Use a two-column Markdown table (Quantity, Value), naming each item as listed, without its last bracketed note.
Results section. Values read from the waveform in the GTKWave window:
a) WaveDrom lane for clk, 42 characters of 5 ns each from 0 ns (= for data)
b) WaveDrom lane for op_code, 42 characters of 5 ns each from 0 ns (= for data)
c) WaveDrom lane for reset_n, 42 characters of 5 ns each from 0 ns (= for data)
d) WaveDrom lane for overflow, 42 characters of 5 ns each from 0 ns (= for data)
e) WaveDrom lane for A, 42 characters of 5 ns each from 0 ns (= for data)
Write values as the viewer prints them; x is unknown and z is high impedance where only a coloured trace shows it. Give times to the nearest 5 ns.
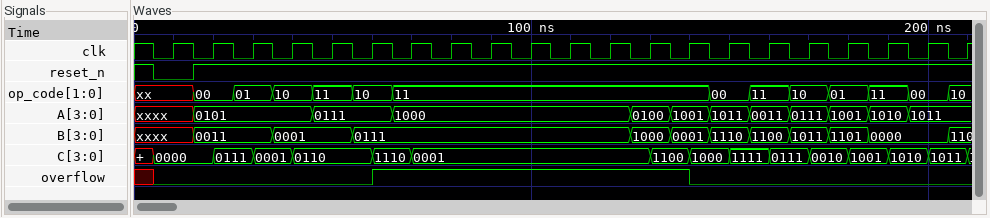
| Quantity | Value |
|---|---|
| WaveDrom lane for clk, 42 characters of 5 ns each from 0 ns | {name: 'clk', wave: '101010101010101010101010101010101010101010'} |
| WaveDrom lane for op_code, 42 characters of 5 ns each from 0 ns | {name: 'op_code', wave: 'x..=.=.=.=.=.=...............=.=.=.=.=.=.=', data: '00 01 10 11 10 11 00 11 10 01 11 00 10'} |
| WaveDrom lane for reset_n, 42 characters of 5 ns each from 0 ns | {name: 'reset_n', wave: '10.1......................................'} |
| WaveDrom lane for overflow, 42 characters of 5 ns each from 0 ns | {name: 'overflow', wave: 'x0..........1...............0.............'} |
| WaveDrom lane for A, 42 characters of 5 ns each from 0 ns | {name: 'A', wave: 'x..=.....=...=...........=.=.=.=.=.=.=.=..', data: '0101 0111 1000 0100 1001 1011 0011 0111 1001 1010 1011'} |
